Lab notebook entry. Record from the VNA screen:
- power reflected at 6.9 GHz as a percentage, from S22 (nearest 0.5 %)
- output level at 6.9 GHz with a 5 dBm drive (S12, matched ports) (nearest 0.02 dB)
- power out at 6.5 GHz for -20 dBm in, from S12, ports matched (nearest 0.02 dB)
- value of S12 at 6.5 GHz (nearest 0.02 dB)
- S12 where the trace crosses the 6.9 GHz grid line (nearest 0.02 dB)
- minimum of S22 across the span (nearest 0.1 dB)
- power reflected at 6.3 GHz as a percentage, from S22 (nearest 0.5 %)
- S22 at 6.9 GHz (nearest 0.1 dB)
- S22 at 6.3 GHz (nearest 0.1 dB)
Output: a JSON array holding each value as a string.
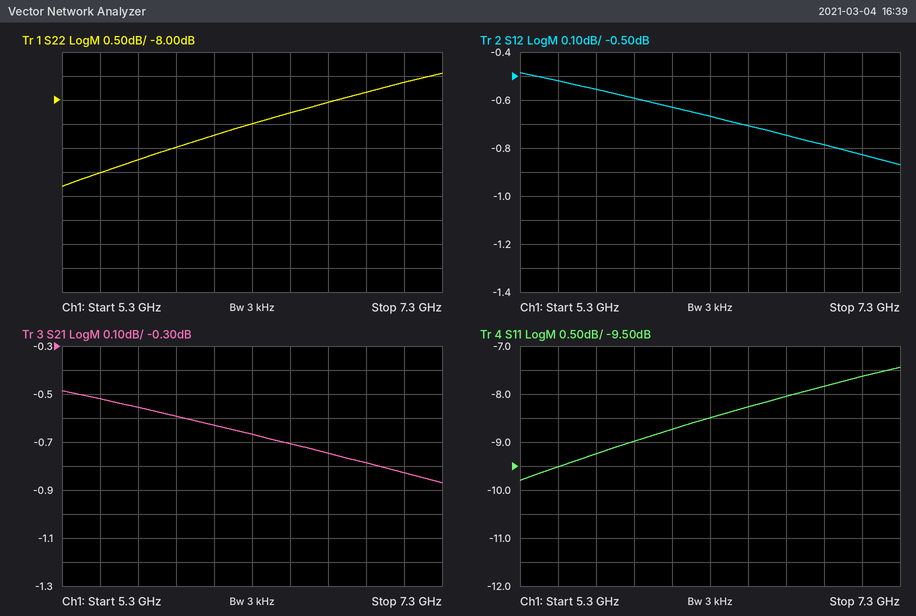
["16.5 %", "4.22 dBm", "-20.70 dBm", "-0.70 dB", "-0.78 dB", "-9.8 dB", "14.0 %", "-7.8 dB", "-8.5 dB"]
